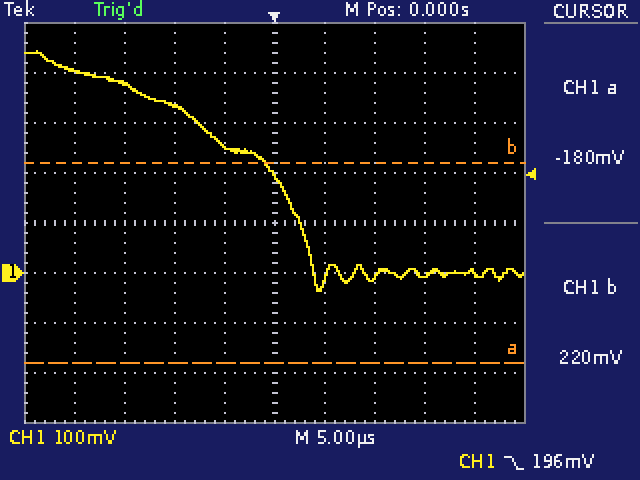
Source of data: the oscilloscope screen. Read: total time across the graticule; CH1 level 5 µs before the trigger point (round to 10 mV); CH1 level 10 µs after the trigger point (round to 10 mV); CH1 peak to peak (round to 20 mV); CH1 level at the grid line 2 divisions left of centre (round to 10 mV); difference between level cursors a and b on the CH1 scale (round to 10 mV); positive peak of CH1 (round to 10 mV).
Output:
50 µs
250 mV
-10 mV
480 mV
340 mV
400 mV
440 mV
